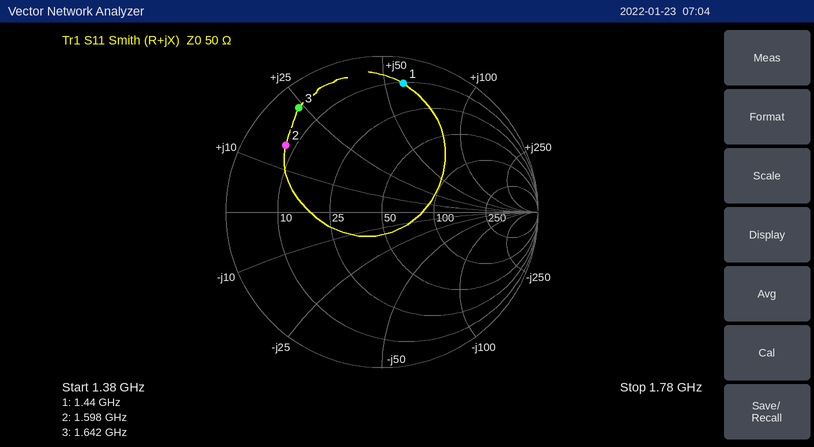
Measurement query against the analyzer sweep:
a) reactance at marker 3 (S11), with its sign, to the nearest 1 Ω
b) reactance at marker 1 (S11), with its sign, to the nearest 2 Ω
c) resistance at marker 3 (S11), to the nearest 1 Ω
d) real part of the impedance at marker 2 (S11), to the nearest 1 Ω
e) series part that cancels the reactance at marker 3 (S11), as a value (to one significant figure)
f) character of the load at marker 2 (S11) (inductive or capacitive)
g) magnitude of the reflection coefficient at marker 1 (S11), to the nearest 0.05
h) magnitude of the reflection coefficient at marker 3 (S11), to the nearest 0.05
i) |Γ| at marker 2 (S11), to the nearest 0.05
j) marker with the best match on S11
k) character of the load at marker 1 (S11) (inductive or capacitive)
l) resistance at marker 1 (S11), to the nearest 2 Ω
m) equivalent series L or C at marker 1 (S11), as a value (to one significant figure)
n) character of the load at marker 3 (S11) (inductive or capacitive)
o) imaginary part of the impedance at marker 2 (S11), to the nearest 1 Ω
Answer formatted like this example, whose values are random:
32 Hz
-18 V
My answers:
+24 Ω
+58 Ω
5 Ω
8 Ω
4 pF
inductive
0.85
0.85
0.75
marker 2
inductive
10 Ω
6 nH
inductive
+15 Ω
